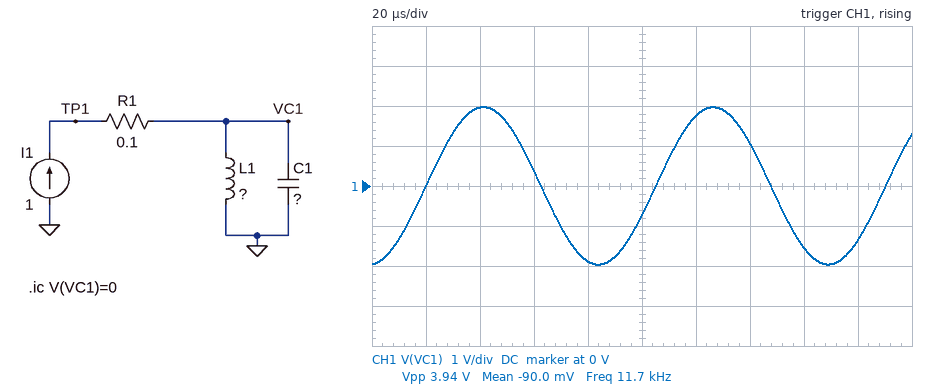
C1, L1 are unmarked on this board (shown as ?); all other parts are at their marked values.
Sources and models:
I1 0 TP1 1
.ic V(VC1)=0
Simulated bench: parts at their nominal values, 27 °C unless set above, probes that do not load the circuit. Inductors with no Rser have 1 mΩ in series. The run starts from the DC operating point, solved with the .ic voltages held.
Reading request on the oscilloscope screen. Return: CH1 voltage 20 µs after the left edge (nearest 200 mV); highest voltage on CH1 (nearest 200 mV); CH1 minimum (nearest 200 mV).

0 V
2.0 V
-2.0 V
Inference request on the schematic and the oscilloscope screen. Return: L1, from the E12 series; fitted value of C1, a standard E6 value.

27 µH
6.8 µF
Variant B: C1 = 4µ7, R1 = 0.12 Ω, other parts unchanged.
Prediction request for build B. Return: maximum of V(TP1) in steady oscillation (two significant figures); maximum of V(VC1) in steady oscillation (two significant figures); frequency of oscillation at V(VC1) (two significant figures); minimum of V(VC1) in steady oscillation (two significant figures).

2.5 V
2.4 V
14 kHz
-2.4 V
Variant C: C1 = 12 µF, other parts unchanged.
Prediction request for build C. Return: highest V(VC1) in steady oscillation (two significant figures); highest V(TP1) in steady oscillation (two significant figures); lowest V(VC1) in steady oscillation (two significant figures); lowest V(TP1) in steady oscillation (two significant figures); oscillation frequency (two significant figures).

1.5 V
1.6 V
-1.5 V
-1.4 V
8.8 kHz
